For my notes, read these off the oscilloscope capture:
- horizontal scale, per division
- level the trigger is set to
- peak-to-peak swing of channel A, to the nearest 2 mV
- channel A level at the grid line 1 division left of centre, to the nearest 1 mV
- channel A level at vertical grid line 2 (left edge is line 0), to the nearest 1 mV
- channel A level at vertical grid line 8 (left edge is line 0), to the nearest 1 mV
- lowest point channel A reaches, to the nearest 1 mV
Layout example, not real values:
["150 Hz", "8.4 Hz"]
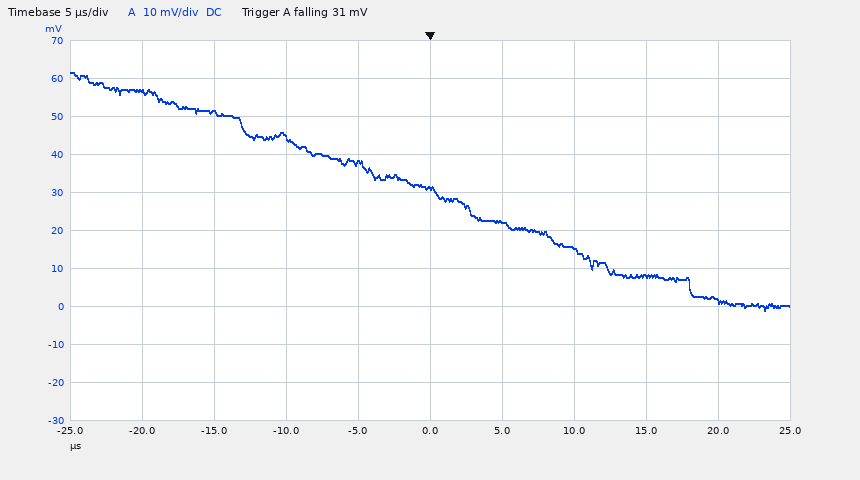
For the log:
["5 µs", "31 mV", "62 mV", "38 mV", "51 mV", "8 mV", "-1 mV"]
